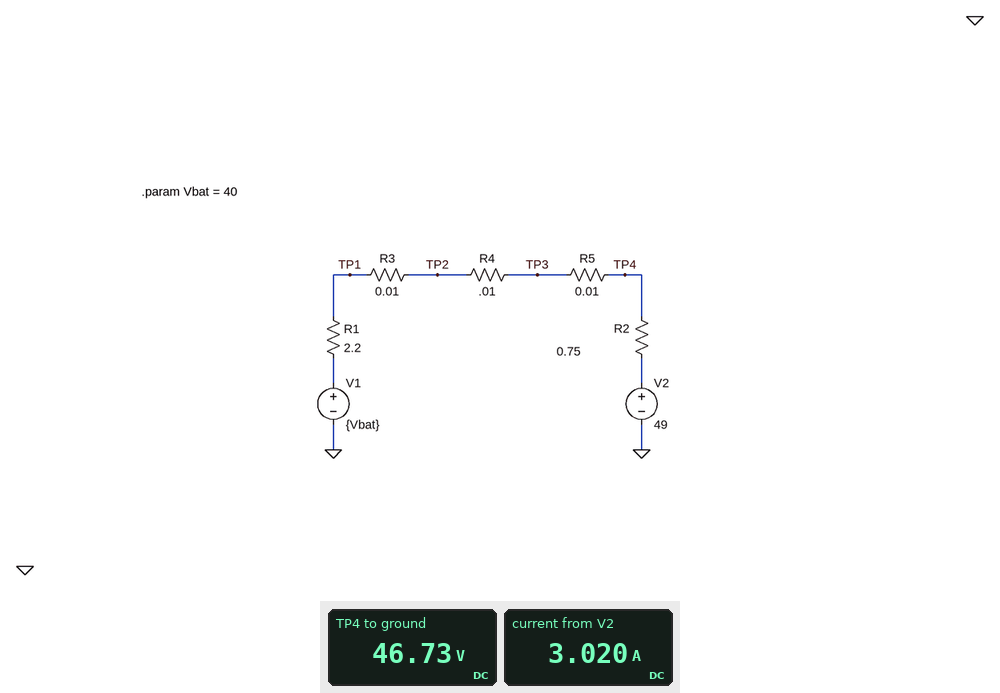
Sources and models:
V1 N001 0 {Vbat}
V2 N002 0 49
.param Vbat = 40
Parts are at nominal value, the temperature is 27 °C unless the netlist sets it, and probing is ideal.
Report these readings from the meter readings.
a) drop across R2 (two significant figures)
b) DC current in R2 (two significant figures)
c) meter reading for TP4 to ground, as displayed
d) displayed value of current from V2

2.3 V
3.0 A
46.73 V
3.020 A
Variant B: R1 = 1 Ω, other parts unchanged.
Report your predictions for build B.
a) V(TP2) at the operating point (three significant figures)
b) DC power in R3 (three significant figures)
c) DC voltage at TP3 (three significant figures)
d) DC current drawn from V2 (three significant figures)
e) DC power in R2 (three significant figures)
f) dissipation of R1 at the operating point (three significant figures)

45.1 V
256 mW
45.2 V
5.06 A
19.2 W
25.6 W
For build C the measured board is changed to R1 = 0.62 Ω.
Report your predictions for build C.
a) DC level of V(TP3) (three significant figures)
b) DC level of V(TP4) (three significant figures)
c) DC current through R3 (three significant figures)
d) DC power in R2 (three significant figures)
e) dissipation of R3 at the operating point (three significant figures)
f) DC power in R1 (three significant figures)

44.1 V
44.2 V
6.43 A
31.0 W
413 mW
25.6 W
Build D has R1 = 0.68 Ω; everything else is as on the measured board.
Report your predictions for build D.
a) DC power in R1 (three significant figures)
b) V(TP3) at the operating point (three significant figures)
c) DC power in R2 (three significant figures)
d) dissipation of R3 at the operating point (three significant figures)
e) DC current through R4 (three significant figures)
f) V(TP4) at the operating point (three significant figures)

25.8 W
44.3 V
28.5 W
380 mW
6.16 A
44.4 V
